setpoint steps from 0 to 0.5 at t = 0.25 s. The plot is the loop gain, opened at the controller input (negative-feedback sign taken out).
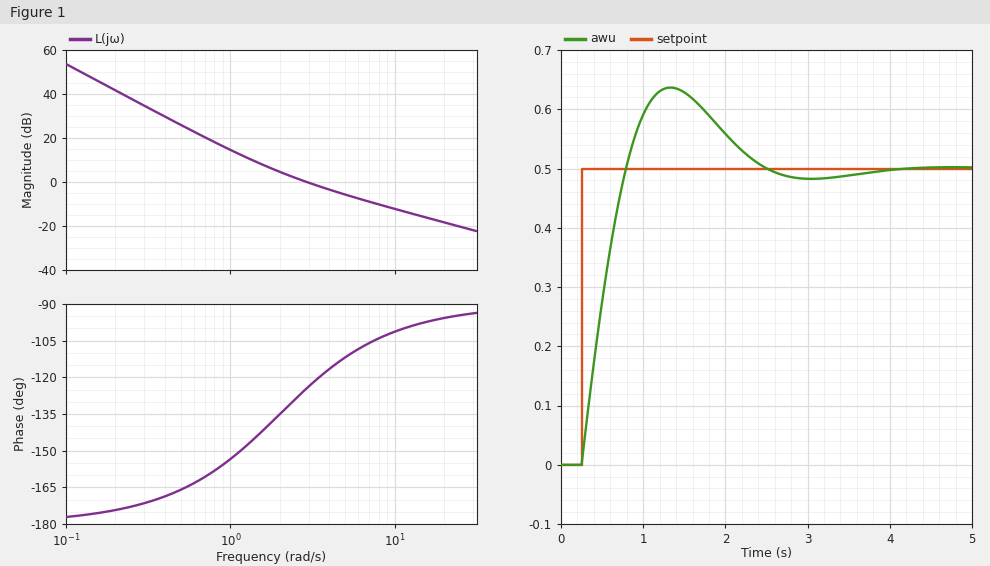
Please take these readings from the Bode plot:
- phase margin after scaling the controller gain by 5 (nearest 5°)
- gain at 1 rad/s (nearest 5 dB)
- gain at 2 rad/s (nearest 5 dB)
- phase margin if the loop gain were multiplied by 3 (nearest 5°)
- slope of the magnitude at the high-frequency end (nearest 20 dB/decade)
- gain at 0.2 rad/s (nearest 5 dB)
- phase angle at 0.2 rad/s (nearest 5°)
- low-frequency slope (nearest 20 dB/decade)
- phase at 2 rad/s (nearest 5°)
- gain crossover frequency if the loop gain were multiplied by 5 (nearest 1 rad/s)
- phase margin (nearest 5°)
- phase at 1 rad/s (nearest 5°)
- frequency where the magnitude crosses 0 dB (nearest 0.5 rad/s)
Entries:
80°
15 dB
5 dB
75°
-20 dB/decade
40 dB
-175°
-40 dB/decade
-135°
12 rad/s
55°
-155°
3.0 rad/s
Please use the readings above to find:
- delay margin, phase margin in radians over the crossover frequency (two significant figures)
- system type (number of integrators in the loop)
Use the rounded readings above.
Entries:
0.32 s
2
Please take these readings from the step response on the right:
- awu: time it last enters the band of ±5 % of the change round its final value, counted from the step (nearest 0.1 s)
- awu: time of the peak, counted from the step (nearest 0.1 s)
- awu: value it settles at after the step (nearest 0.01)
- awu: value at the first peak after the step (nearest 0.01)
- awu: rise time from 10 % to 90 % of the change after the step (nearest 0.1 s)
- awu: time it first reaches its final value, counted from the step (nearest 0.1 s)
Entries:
2.0 s
1.1 s
0.50
0.64
0.4 s
0.5 s
